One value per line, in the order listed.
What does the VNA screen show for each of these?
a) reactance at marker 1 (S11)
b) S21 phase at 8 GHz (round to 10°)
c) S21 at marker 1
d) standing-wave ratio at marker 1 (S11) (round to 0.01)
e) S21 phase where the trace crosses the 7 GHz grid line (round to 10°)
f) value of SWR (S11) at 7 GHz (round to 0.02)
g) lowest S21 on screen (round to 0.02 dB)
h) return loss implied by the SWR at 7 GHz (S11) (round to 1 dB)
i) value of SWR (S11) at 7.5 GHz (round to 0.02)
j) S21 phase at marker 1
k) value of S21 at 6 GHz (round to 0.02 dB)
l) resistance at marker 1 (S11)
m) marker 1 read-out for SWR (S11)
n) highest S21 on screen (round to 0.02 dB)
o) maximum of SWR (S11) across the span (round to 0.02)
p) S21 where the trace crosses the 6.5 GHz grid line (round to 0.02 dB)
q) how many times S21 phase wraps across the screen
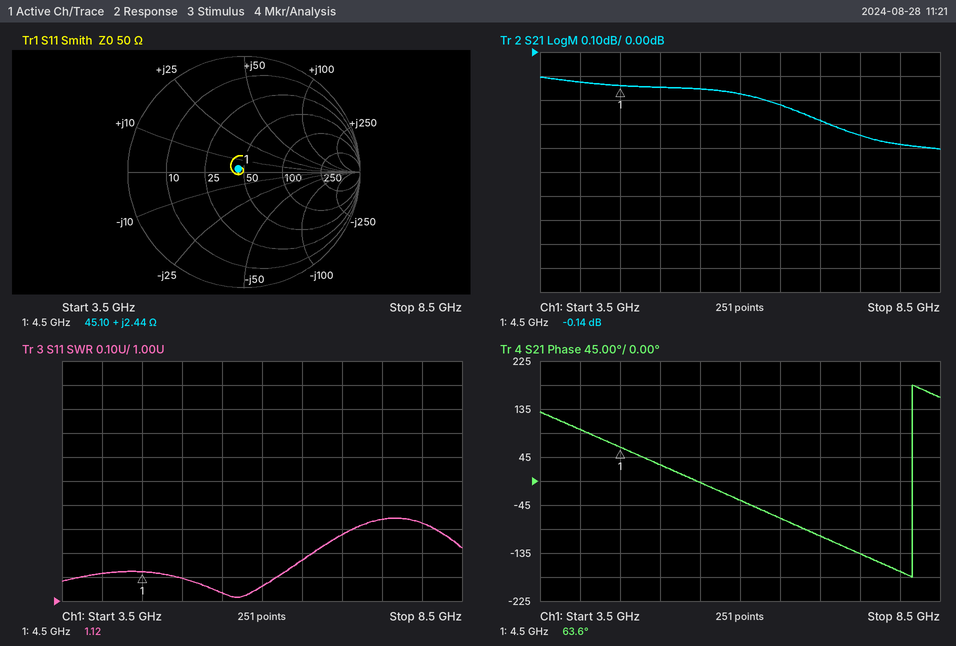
+2.44 Ω
-170°
-0.14 dB
1.12
-100°
1.28
-0.40 dB
18 dB
1.34
63.6°
-0.18 dB
45.10 Ω
1.12
-0.10 dB
1.34
-0.22 dB
1
